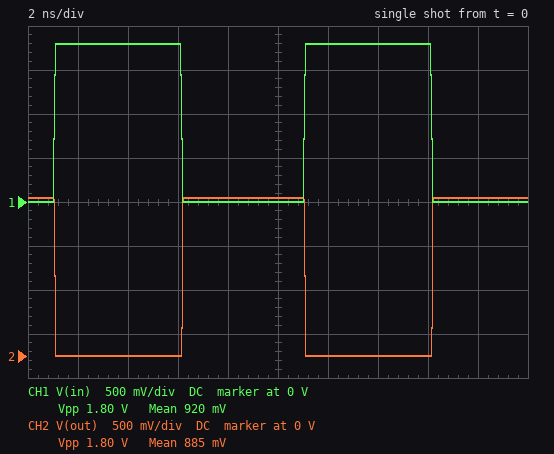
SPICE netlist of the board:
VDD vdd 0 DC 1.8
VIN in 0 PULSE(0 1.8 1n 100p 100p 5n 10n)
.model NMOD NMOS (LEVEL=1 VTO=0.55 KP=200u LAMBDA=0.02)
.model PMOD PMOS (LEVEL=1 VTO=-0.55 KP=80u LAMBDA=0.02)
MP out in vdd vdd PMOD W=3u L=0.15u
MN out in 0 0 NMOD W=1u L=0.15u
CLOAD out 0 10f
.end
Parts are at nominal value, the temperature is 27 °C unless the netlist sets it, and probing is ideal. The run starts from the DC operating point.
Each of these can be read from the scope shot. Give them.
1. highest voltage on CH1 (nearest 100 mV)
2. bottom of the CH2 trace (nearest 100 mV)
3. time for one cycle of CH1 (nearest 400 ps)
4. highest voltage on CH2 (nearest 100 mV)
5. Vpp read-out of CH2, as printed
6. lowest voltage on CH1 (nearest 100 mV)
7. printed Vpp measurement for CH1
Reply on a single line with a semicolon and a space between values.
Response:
1.8 V; 0 V; 10.0 ns; 1.8 V; 1.80 V; 0 V; 1.80 V
